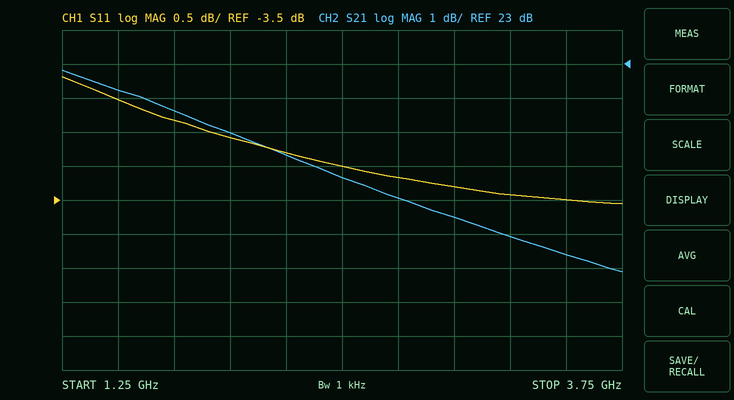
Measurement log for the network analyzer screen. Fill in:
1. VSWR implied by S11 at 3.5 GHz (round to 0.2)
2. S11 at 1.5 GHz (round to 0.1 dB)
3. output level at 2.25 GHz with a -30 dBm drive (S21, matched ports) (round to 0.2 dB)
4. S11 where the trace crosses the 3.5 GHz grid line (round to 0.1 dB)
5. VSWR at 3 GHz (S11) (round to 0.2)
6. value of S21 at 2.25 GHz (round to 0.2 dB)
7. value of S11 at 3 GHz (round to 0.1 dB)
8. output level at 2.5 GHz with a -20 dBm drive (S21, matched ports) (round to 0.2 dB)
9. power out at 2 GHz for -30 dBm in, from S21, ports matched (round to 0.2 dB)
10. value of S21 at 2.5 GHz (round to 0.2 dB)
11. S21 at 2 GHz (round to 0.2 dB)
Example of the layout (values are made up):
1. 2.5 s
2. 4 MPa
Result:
1. 5.0
2. -2.0 dB
3. -9.6 dBm
4. -3.5 dB
5. 5.4
6. 20.4 dB
7. -3.3 dB
8. -0.4 dBm
9. -9.0 dBm
10. 19.6 dB
11. 21.0 dB
